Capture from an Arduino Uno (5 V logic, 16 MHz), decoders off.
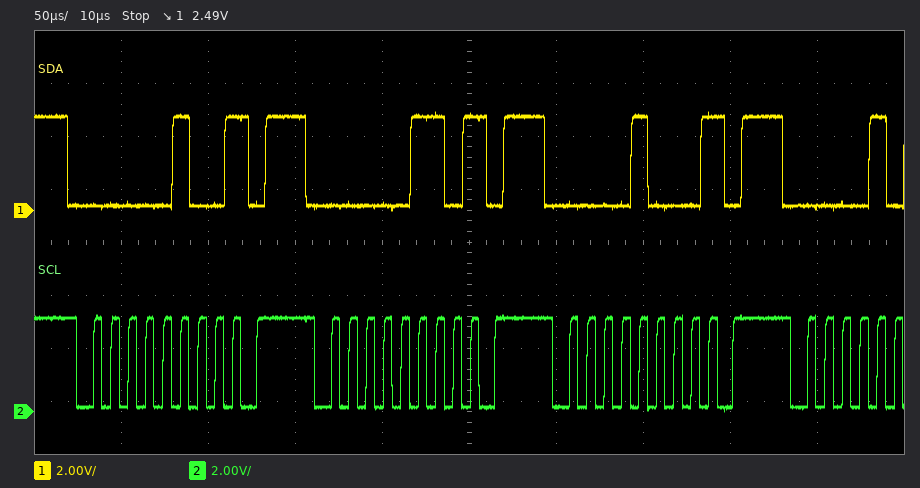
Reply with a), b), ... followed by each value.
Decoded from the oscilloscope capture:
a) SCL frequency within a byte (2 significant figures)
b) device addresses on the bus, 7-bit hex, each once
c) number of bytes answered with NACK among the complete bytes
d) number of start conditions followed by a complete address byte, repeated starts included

a) 100 kHz
b) 0x02 0x03 0x04
c) 3
d) 3
